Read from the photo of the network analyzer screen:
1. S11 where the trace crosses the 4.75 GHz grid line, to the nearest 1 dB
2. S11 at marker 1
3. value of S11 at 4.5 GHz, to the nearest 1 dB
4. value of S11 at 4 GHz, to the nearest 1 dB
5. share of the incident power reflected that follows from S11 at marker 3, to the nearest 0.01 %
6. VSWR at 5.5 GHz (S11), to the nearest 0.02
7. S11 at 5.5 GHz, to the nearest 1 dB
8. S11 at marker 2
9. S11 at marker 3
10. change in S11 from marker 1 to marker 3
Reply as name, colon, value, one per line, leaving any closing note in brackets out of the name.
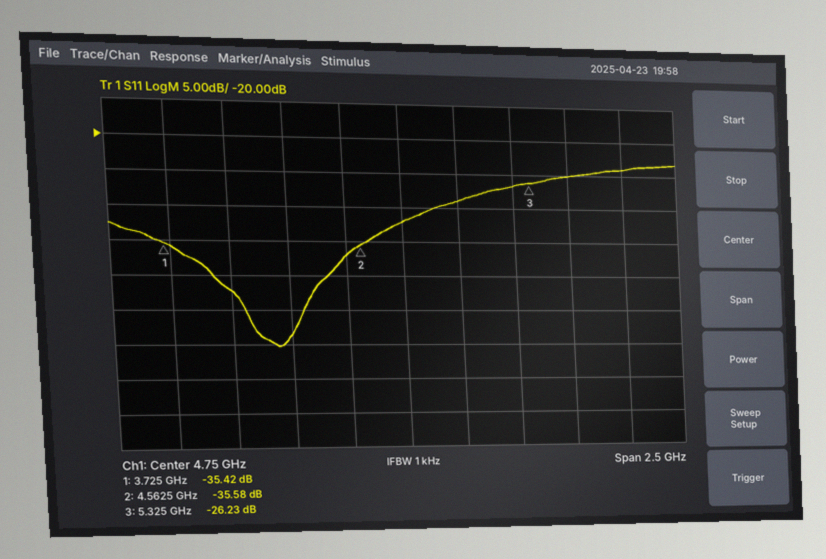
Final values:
S11 where the trace crosses the 4.75 GHz grid line, to the nearest 1 dB: -32 dB
S11 at marker 1: -35.42 dB
value of S11 at 4.5 GHz, to the nearest 1 dB: -37 dB
value of S11 at 4 GHz, to the nearest 1 dB: -42 dB
share of the incident power reflected that follows from S11 at marker 3, to the nearest 0.01 %: 0.24 %
VSWR at 5.5 GHz (S11), to the nearest 0.02: 1.12
S11 at 5.5 GHz, to the nearest 1 dB: -25 dB
S11 at marker 2: -35.58 dB
S11 at marker 3: -26.23 dB
change in S11 from marker 1 to marker 3: 9.19 dB
